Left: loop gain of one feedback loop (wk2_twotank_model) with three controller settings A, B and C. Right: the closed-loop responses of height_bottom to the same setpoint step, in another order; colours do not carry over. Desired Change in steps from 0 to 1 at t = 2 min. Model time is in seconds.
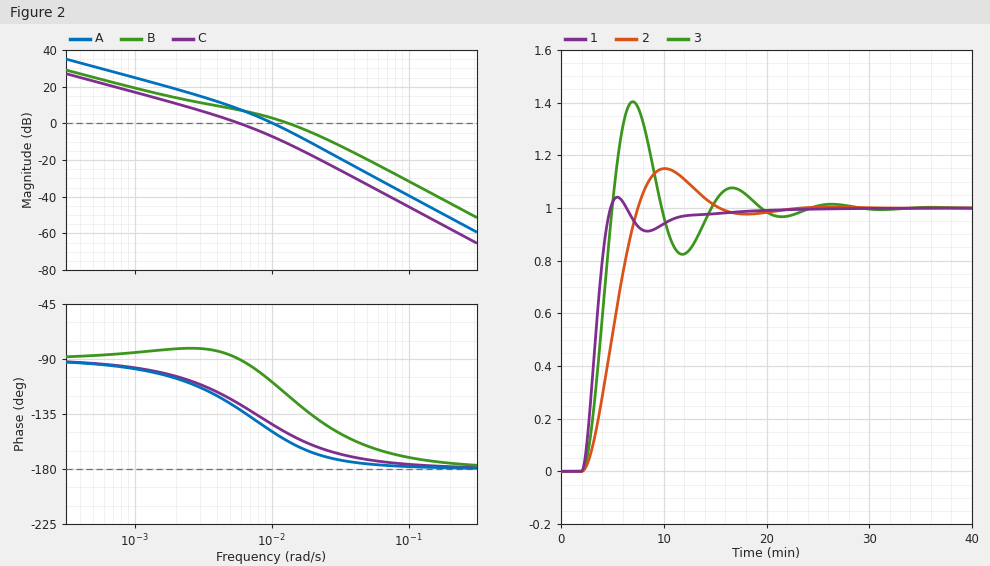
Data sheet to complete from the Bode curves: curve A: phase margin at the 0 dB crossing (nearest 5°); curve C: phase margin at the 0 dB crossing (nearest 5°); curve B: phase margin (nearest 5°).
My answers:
30°
55°
60°
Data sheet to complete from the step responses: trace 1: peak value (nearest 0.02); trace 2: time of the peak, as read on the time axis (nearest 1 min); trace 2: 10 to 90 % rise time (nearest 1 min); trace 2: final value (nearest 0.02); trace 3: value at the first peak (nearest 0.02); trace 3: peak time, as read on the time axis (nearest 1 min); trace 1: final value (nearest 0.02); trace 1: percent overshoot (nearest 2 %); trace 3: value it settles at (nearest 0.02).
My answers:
1.04
10 min
4 min
1.00
1.40
7 min
1.00
4 %
1.00
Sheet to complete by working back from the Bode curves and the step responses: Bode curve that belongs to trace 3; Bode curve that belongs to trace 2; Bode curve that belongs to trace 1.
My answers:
A
C
B
